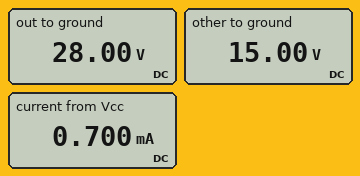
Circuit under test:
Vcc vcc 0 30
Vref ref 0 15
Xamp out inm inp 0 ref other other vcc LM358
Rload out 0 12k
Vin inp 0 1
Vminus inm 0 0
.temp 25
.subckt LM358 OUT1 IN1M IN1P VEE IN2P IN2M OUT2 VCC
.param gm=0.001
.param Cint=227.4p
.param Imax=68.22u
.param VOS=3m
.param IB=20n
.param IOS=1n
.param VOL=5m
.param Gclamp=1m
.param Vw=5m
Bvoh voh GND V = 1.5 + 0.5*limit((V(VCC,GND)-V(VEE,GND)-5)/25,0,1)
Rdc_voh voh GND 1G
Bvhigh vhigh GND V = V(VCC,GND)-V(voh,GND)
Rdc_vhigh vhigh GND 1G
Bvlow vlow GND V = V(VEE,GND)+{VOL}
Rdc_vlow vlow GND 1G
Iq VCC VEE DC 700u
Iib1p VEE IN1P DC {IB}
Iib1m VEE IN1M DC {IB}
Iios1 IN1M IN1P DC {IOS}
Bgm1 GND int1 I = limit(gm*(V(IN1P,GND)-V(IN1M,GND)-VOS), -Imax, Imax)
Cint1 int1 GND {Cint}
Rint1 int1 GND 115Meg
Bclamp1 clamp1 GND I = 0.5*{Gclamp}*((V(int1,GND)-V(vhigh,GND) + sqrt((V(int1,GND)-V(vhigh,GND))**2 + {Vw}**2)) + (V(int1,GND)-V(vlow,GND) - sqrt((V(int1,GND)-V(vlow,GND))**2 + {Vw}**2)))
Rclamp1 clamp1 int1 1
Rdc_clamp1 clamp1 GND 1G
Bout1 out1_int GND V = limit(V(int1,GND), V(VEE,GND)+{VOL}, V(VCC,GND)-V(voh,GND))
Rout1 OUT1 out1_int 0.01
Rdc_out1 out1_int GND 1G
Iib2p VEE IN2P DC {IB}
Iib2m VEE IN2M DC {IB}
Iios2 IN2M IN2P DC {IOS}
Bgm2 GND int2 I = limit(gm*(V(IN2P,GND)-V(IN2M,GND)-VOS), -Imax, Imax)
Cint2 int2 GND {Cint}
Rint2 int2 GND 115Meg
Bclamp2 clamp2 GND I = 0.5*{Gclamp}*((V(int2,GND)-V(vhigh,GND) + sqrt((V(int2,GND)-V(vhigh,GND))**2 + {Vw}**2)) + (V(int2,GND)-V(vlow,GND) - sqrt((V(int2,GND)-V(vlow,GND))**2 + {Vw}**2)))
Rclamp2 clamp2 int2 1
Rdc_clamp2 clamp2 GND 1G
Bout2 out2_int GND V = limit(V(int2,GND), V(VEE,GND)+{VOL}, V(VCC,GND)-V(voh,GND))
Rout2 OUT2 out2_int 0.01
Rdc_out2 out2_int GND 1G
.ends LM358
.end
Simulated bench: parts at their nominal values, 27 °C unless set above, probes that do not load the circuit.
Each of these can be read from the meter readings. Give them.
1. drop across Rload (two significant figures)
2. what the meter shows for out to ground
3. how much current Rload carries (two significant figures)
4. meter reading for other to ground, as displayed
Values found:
28 V
28.00 V
2.3 mA
15.00 V
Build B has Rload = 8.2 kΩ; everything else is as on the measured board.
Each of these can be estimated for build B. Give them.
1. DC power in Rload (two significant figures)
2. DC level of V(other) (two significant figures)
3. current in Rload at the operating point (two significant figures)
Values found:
96 mW
15 V
3.4 mA
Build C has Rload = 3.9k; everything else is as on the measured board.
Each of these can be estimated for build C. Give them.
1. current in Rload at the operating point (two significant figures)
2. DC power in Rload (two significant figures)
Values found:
7.2 mA
200 mW
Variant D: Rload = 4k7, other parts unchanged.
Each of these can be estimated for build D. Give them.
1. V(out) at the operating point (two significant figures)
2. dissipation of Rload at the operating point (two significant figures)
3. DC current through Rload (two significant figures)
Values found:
28 V
170 mW
6.0 mA
